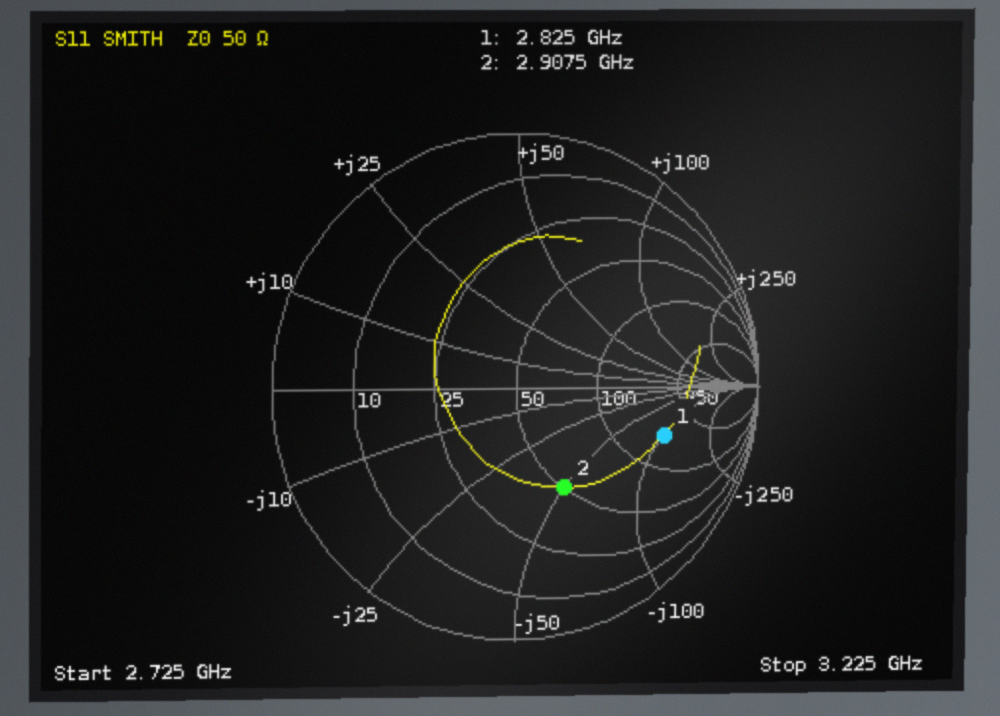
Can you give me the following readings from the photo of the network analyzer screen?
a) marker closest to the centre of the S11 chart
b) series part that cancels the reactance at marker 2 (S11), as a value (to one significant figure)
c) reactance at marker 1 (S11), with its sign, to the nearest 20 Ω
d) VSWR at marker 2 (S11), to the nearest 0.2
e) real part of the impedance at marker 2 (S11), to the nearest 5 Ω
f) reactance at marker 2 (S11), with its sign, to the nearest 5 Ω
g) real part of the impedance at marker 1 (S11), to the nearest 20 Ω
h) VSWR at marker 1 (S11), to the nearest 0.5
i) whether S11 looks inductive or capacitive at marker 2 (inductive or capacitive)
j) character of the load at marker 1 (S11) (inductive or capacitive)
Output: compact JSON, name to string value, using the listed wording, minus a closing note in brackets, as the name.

{"marker closest to the centre of the S11 chart": "marker 2", "series part that cancels the reactance at marker 2 (S11), as a value": "3 nH", "reactance at marker 1 (S11), with its sign, to the nearest 20 Ω": "-100 Ω", "VSWR at marker 2 (S11), to the nearest 0.2": "2.6", "real part of the impedance at marker 2 (S11), to the nearest 5 Ω": "50 Ω", "reactance at marker 2 (S11), with its sign, to the nearest 5 Ω": "-50 Ω", "real part of the impedance at marker 1 (S11), to the nearest 20 Ω": "160 Ω", "VSWR at marker 1 (S11), to the nearest 0.5": "4.5", "whether S11 looks inductive or capacitive at marker 2": "capacitive", "character of the load at marker 1 (S11)": "capacitive"}
